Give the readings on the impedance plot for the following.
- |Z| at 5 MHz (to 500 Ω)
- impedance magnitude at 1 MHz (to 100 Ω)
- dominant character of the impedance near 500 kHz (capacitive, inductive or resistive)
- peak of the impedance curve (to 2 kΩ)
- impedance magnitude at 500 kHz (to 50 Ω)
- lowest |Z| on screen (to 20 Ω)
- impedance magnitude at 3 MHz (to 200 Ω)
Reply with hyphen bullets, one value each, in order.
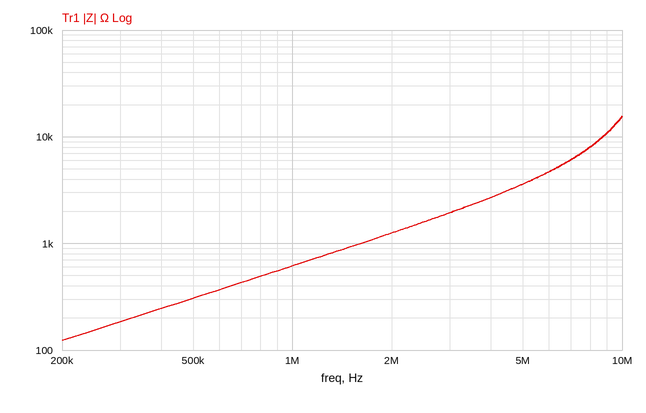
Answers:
- 3.5 kΩ
- 600 Ω
- inductive
- 16 kΩ
- 300 Ω
- 120 Ω
- 2.0 kΩ
